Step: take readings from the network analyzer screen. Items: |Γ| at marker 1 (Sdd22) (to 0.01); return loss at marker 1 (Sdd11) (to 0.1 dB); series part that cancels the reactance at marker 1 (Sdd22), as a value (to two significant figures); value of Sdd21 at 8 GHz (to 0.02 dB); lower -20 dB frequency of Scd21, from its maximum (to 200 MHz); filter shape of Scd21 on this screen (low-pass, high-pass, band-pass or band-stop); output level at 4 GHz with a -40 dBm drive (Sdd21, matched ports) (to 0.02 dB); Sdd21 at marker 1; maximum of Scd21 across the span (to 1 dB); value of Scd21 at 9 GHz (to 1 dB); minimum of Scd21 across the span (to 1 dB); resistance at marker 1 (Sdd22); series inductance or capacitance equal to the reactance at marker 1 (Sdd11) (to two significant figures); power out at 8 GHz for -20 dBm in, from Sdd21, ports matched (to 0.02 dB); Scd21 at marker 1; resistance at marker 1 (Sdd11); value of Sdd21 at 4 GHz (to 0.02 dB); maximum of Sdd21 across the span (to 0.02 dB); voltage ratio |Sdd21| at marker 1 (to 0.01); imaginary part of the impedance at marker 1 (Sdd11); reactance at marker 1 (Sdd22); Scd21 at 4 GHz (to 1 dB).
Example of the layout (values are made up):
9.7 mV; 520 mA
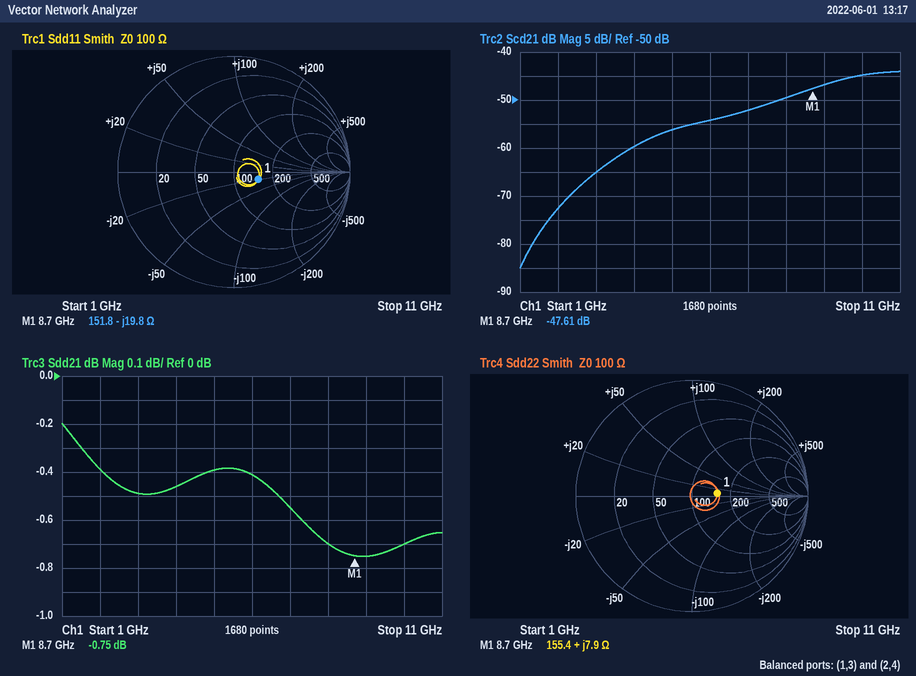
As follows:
0.22; 13.2 dB; 2.3 pF; -0.70 dB; 3.2 GHz; high-pass; -40.46 dBm; -0.75 dB; -44 dB; -47 dB; -85 dB; 155.4 Ω; 920 fF; -20.70 dBm; -47.61 dB; 151.8 Ω; -0.46 dB; -0.20 dB; 0.92; -19.8 Ω; +7.9 Ω; -60 dB
